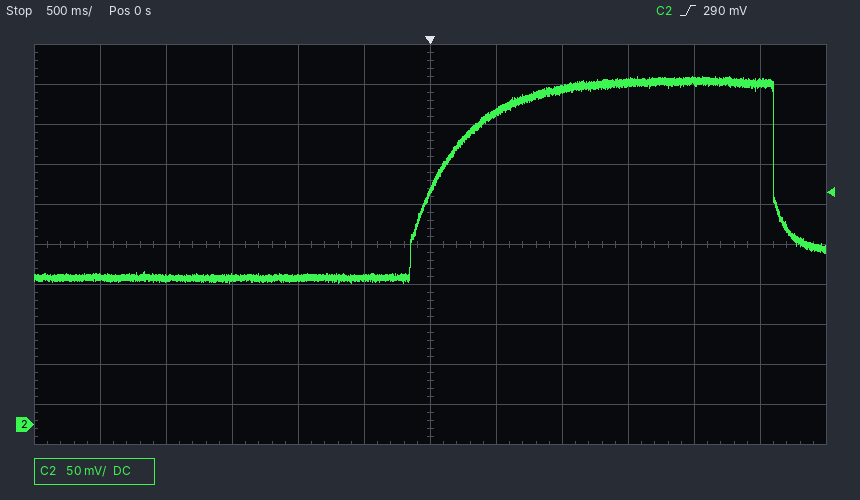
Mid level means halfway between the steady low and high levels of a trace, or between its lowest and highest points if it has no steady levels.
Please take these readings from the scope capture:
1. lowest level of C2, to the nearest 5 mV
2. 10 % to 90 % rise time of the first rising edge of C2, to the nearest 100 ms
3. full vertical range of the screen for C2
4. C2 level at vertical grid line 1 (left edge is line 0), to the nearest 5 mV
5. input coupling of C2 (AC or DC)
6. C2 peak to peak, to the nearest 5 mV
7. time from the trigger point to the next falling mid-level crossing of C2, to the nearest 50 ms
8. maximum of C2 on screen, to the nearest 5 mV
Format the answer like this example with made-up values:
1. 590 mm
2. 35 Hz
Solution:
1. 175 mV
2. 800 ms
3. 500 mV
4. 185 mV
5. DC
6. 260 mV
7. 2.60 s
8. 435 mV
